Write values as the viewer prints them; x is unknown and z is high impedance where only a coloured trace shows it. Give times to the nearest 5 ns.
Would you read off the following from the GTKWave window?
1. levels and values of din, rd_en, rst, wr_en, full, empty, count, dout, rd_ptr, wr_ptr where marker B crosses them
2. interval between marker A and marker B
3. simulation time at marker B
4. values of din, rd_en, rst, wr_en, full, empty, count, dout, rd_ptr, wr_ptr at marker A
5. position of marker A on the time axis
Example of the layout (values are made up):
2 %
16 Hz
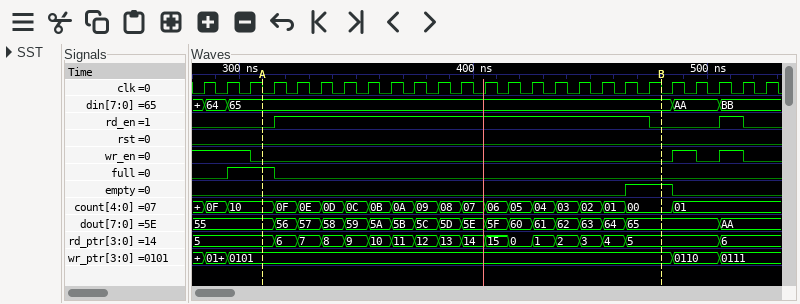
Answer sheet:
din=65, rd_en=0, rst=0, wr_en=0, full=0, empty=1, count=00, dout=65, rd_ptr=5, wr_ptr=0101
170 ns
480 ns
din=65, rd_en=0, rst=0, wr_en=0, full=1, empty=0, count=10, dout=55, rd_ptr=5, wr_ptr=0101
310 ns
